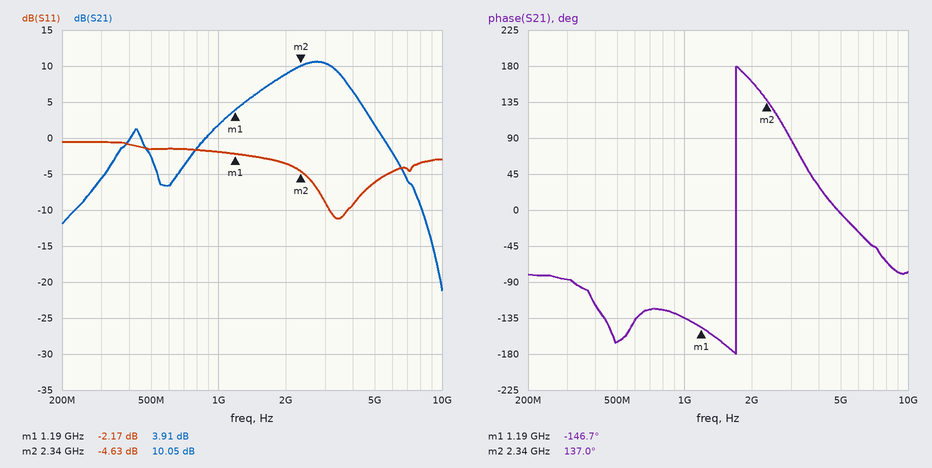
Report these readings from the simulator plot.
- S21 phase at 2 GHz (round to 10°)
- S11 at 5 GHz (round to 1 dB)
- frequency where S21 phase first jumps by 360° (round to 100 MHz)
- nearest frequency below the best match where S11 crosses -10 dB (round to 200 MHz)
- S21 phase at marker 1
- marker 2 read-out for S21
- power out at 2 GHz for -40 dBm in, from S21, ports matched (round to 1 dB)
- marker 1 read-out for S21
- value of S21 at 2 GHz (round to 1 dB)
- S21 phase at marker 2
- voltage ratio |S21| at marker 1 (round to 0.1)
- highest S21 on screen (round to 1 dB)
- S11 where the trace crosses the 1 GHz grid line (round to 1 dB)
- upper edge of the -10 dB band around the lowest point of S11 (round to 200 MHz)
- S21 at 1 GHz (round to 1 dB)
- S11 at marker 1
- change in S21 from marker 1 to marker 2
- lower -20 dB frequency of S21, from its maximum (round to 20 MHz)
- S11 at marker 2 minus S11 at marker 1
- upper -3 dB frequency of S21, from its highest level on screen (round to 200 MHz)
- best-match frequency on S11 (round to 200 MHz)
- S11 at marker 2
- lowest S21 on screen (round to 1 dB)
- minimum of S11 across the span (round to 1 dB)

160°
-6 dB
1.7 GHz
3.2 GHz
-146.7°
10.05 dB
-31 dBm
3.91 dB
9 dB
137.0°
1.6
11 dB
-2 dB
3.8 GHz
2 dB
-2.17 dB
6.14 dB
240 MHz
-2.46 dB
3.8 GHz
3.4 GHz
-4.63 dB
-21 dB
-11 dB
